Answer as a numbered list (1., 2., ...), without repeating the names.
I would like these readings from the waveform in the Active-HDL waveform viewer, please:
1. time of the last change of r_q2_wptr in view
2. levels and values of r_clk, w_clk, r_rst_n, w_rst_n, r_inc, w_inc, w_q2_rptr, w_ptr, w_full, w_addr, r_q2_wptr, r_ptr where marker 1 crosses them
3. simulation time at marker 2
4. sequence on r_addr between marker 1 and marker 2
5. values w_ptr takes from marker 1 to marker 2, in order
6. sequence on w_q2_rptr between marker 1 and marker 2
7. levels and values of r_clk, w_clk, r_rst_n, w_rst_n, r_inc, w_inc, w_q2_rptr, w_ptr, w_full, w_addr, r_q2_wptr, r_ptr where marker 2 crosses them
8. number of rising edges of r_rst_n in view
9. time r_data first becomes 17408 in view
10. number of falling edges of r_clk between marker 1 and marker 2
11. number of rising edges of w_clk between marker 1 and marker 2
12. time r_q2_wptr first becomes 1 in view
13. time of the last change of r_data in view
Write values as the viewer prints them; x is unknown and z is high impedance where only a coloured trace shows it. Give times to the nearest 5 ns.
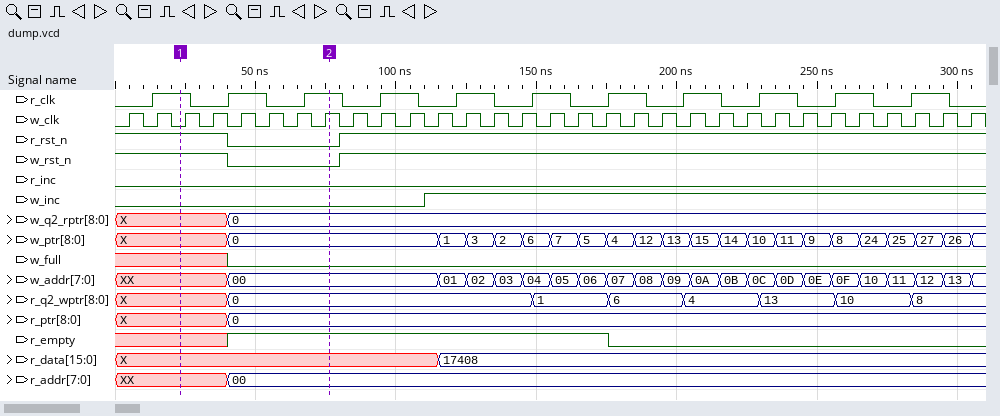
1. 285 ns
2. r_clk=1, w_clk=0, r_rst_n=1, w_rst_n=1, r_inc=0, w_inc=0, w_q2_rptr=X, w_ptr=X, w_full=x, w_addr=XX, r_q2_wptr=X, r_ptr=X
3. 75 ns
4. XX, 00
5. X, 0
6. X, 0
7. r_clk=1, w_clk=1, r_rst_n=0, w_rst_n=0, r_inc=0, w_inc=0, w_q2_rptr=0, w_ptr=0, w_full=0, w_addr=00, r_q2_wptr=0, r_ptr=0
8. 1
9. 115 ns
10. 2
11. 6
12. 150 ns
13. 115 ns
